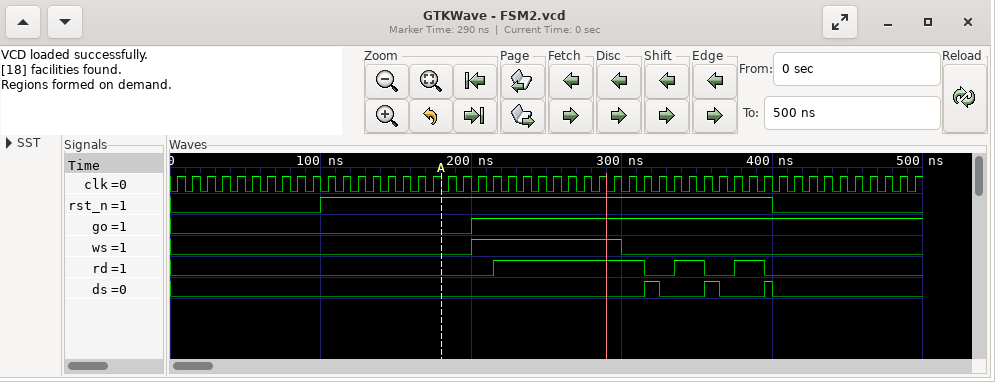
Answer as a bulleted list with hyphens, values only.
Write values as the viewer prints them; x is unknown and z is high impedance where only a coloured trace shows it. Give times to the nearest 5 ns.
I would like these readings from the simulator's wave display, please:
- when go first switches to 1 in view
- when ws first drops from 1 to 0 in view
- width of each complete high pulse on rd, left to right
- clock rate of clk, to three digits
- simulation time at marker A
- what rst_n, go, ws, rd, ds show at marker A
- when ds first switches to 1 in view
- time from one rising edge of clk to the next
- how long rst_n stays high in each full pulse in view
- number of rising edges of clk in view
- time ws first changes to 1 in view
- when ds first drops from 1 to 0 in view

- 200 ns
- 300 ns
- 100 ns, 20 ns, 20 ns
- 100 MHz
- 180 ns
- rst_n=1, go=0, ws=0, rd=0, ds=0
- 315 ns
- 10 ns
- 300 ns
- 50
- 200 ns
- 325 ns
